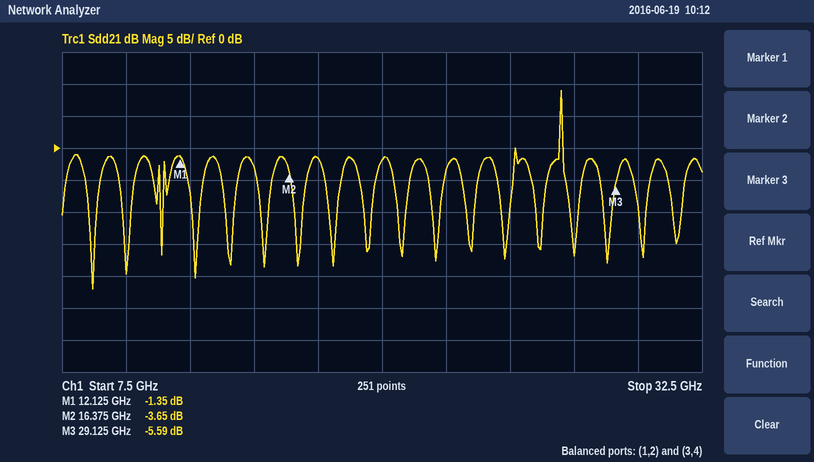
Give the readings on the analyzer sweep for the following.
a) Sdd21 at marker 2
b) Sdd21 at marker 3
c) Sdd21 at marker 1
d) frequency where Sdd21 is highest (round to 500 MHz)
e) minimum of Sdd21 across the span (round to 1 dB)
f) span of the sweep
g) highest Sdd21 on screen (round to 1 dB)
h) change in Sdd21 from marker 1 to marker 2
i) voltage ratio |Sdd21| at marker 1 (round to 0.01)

-3.65 dB
-5.59 dB
-1.35 dB
27.0 GHz
-22 dB
25 GHz
9 dB
-2.30 dB
0.86
